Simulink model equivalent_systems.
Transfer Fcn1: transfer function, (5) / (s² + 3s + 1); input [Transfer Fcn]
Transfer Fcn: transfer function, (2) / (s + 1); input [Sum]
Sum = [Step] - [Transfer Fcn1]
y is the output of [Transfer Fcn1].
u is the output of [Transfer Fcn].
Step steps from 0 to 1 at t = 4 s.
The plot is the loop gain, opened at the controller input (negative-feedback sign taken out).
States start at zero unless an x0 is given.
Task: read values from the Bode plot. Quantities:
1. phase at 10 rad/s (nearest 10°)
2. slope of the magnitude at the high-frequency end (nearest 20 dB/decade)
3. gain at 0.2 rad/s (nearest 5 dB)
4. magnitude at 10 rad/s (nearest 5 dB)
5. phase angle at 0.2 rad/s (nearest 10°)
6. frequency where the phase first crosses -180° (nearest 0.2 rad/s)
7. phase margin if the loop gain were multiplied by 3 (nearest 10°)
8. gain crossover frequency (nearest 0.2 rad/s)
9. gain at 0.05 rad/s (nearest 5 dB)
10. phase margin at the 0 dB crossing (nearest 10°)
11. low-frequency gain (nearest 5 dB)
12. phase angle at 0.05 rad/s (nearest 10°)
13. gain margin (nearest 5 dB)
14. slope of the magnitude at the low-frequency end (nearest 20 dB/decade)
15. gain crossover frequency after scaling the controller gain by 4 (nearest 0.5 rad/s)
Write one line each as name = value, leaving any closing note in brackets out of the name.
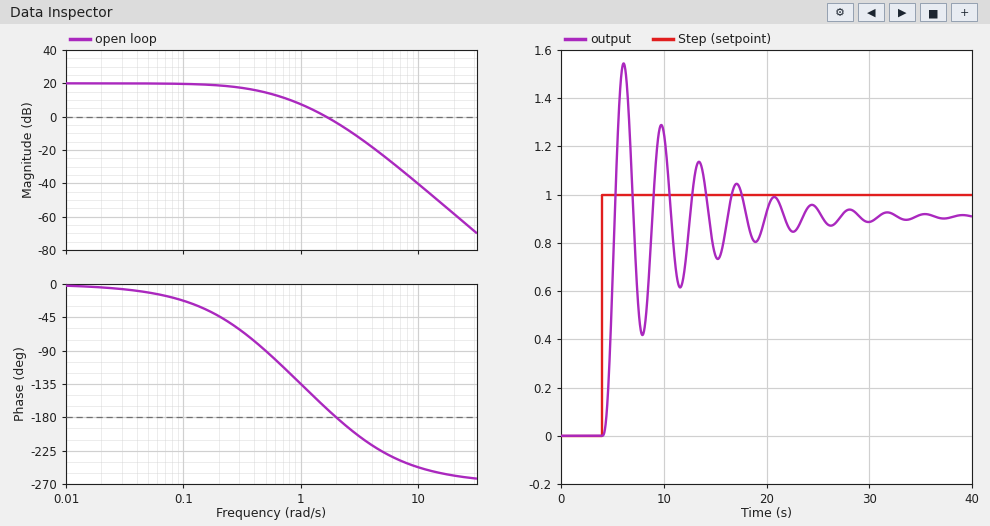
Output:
phase at 10 rad/s = -250°
slope of the magnitude at the high-frequency end = -60 dB/decade
gain at 0.2 rad/s = 20 dB
magnitude at 10 rad/s = -40 dB
phase angle at 0.2 rad/s = -40°
frequency where the phase first crosses -180° = 2.0 rad/s
phase margin if the loop gain were multiplied by 3 = -20°
gain crossover frequency = 1.6 rad/s
gain at 0.05 rad/s = 20 dB
phase margin at the 0 dB crossing = 10°
low-frequency gain = 20 dB
phase angle at 0.05 rad/s = -10°
gain margin = 5 dB
slope of the magnitude at the low-frequency end = 0 dB/decade
gain crossover frequency after scaling the controller gain by 4 = 3.0 rad/s
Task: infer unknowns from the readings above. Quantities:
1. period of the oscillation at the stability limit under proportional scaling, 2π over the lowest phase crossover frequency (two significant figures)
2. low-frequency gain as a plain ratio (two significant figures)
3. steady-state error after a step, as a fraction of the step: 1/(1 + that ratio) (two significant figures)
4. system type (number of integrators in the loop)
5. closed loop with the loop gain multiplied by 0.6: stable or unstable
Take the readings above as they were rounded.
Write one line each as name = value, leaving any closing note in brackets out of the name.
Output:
period of the oscillation at the stability limit under proportional scaling, 2π over the lowest phase crossover frequency = 3.1 s
low-frequency gain as a plain ratio = 10
steady-state error after a step, as a fraction of the step: 1/(1 + that ratio) = 0.091
system type = 0
closed loop with the loop gain multiplied by 0.6: stable or unstable = stable
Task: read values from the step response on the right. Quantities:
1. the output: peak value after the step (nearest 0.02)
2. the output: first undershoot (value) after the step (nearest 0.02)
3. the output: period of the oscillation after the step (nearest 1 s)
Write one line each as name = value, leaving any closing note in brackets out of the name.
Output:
the output: peak value after the step = 1.54
the output: first undershoot (value) after the step = 0.42
the output: period of the oscillation after the step = 4 s
